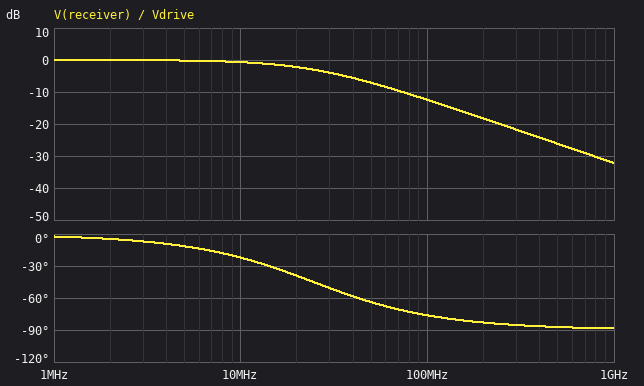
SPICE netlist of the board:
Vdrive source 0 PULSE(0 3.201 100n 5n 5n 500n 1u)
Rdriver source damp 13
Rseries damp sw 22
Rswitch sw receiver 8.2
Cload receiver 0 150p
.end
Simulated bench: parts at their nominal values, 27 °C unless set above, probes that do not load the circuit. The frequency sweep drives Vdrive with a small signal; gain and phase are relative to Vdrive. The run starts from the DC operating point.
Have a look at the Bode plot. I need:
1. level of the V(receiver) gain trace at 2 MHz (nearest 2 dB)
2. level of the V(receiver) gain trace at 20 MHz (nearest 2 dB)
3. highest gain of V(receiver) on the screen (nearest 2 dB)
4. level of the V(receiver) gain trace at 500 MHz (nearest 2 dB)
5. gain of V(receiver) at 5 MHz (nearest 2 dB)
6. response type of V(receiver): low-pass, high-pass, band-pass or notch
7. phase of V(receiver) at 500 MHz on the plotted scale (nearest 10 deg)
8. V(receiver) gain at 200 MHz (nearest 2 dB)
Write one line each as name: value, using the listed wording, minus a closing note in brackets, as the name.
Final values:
level of the V(receiver) gain trace at 2 MHz: 0 dB
level of the V(receiver) gain trace at 20 MHz: -2 dB
highest gain of V(receiver) on the screen: 0 dB
level of the V(receiver) gain trace at 500 MHz: -26 dB
gain of V(receiver) at 5 MHz: 0 dB
response type of V(receiver): low-pass, high-pass, band-pass or notch: low-pass
phase of V(receiver) at 500 MHz on the plotted scale: -90 deg
V(receiver) gain at 200 MHz: -18 dB
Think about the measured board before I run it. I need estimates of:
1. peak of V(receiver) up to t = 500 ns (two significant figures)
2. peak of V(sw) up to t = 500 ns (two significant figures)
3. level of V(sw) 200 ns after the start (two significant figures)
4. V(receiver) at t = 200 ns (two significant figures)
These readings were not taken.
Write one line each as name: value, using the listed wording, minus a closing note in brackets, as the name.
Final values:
peak of V(receiver) up to t = 500 ns: 3.2 V
peak of V(sw) up to t = 500 ns: 3.2 V
level of V(sw) 200 ns after the start: 3.2 V
V(receiver) at t = 200 ns: 3.2 V
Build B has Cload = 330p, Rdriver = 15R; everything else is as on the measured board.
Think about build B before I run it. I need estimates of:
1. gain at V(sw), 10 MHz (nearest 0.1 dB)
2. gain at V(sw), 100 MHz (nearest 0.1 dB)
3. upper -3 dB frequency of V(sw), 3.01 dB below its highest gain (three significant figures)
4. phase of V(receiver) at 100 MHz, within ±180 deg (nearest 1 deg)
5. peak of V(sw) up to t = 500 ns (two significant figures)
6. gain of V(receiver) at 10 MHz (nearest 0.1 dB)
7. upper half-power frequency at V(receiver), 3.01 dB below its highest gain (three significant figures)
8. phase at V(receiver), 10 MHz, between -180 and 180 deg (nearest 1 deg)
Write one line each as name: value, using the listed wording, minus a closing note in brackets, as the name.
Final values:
gain at V(sw), 10 MHz: -2.6 dB
gain at V(sw), 100 MHz: -13.6 dB
upper -3 dB frequency of V(sw), 3.01 dB below its highest gain: 11.0 MHz
phase of V(receiver) at 100 MHz, within ±180 deg: -84 deg
peak of V(sw) up to t = 500 ns: 3.2 V
gain of V(receiver) at 10 MHz: -2.7 dB
upper half-power frequency at V(receiver), 3.01 dB below its highest gain: 10.7 MHz
phase at V(receiver), 10 MHz, between -180 and 180 deg: -43 deg
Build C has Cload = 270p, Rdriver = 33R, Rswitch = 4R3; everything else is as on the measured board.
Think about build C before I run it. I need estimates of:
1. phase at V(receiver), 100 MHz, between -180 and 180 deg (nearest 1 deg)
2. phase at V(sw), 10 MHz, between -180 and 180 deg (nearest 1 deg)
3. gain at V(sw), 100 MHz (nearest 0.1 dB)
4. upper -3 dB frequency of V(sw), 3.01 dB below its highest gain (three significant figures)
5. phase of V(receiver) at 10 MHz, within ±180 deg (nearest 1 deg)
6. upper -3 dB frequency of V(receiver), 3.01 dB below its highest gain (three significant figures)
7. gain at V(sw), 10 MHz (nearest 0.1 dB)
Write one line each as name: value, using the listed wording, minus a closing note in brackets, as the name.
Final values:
phase at V(receiver), 100 MHz, between -180 and 180 deg: -84 deg
phase at V(sw), 10 MHz, between -180 and 180 deg: -41 deg
gain at V(sw), 100 MHz: -18.2 dB
upper -3 dB frequency of V(sw), 3.01 dB below its highest gain: 9.99 MHz
phase of V(receiver) at 10 MHz, within ±180 deg: -45 deg
upper -3 dB frequency of V(receiver), 3.01 dB below its highest gain: 9.94 MHz
gain at V(sw), 10 MHz: -3.0 dB
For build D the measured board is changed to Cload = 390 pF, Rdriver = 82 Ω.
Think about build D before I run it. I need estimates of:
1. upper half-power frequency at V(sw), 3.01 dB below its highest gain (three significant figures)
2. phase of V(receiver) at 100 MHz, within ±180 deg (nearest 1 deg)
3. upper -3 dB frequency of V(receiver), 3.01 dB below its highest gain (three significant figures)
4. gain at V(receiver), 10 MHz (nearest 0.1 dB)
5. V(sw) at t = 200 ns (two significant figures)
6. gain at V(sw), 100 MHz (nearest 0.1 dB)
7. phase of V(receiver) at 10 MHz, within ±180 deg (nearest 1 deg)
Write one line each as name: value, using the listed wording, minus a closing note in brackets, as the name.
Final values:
upper half-power frequency at V(sw), 3.01 dB below its highest gain: 3.66 MHz
phase of V(receiver) at 100 MHz, within ±180 deg: -88 deg
upper -3 dB frequency of V(receiver), 3.01 dB below its highest gain: 3.64 MHz
gain at V(receiver), 10 MHz: -9.3 dB
V(sw) at t = 200 ns: 2.9 V
gain at V(sw), 100 MHz: -21.8 dB
phase of V(receiver) at 10 MHz, within ±180 deg: -70 deg
